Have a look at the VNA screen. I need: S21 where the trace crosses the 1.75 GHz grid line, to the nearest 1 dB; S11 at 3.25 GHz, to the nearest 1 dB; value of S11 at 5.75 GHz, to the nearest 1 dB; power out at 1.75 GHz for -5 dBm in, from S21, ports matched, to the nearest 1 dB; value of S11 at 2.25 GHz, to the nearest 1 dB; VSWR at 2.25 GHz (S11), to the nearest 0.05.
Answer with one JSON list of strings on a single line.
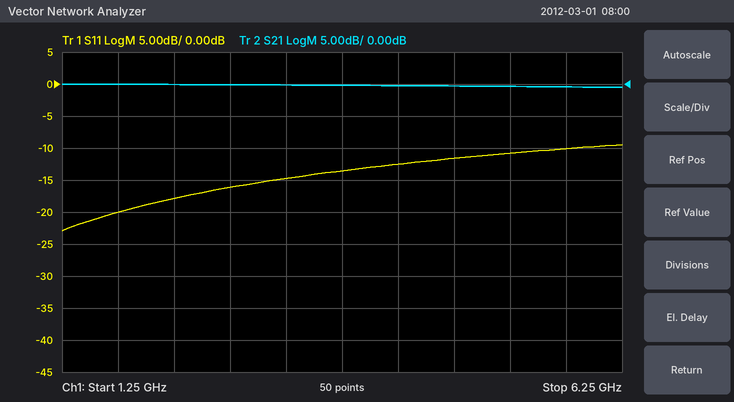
["0 dB", "-15 dB", "-10 dB", "-5 dBm", "-18 dB", "1.30"]
